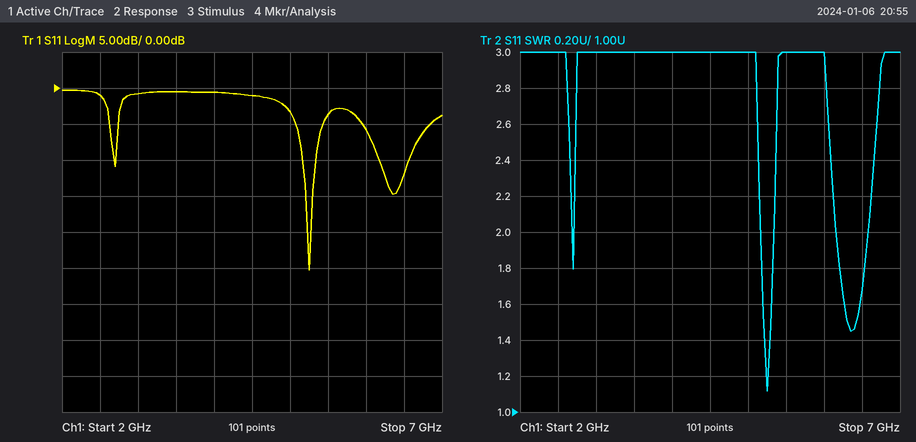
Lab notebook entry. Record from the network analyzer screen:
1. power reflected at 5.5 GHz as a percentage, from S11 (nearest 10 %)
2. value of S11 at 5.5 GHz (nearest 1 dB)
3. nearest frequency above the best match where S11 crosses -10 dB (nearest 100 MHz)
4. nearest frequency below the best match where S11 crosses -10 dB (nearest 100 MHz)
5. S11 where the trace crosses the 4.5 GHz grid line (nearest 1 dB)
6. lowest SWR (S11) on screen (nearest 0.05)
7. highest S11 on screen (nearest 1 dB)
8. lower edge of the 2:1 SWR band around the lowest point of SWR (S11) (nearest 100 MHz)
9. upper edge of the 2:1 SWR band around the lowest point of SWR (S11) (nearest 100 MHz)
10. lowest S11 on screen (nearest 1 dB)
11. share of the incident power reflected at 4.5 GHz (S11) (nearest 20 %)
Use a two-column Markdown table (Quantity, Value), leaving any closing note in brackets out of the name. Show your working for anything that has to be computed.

| Quantity | Value |
|---|---|
| power reflected at 5.5 GHz as a percentage, from S11 | 10^(-4/10) ≈ 40 % |
| value of S11 at 5.5 GHz | -4 dB |
| nearest frequency above the best match where S11 crosses -10 dB | 5.3 GHz |
| nearest frequency below the best match where S11 crosses -10 dB | 5.2 GHz |
| S11 where the trace crosses the 4.5 GHz grid line | -1 dB |
| lowest SWR (S11) on screen | 1.10 |
| highest S11 on screen | 0 dB |
| lower edge of the 2:1 SWR band around the lowest point of SWR (S11) | 5.2 GHz |
| upper edge of the 2:1 SWR band around the lowest point of SWR (S11) | 5.3 GHz |
| lowest S11 on screen | -25 dB |
| share of the incident power reflected at 4.5 GHz (S11) | 10^(-1/10) ≈ 79.4 %, so 80 % to the nearest 20 % |
